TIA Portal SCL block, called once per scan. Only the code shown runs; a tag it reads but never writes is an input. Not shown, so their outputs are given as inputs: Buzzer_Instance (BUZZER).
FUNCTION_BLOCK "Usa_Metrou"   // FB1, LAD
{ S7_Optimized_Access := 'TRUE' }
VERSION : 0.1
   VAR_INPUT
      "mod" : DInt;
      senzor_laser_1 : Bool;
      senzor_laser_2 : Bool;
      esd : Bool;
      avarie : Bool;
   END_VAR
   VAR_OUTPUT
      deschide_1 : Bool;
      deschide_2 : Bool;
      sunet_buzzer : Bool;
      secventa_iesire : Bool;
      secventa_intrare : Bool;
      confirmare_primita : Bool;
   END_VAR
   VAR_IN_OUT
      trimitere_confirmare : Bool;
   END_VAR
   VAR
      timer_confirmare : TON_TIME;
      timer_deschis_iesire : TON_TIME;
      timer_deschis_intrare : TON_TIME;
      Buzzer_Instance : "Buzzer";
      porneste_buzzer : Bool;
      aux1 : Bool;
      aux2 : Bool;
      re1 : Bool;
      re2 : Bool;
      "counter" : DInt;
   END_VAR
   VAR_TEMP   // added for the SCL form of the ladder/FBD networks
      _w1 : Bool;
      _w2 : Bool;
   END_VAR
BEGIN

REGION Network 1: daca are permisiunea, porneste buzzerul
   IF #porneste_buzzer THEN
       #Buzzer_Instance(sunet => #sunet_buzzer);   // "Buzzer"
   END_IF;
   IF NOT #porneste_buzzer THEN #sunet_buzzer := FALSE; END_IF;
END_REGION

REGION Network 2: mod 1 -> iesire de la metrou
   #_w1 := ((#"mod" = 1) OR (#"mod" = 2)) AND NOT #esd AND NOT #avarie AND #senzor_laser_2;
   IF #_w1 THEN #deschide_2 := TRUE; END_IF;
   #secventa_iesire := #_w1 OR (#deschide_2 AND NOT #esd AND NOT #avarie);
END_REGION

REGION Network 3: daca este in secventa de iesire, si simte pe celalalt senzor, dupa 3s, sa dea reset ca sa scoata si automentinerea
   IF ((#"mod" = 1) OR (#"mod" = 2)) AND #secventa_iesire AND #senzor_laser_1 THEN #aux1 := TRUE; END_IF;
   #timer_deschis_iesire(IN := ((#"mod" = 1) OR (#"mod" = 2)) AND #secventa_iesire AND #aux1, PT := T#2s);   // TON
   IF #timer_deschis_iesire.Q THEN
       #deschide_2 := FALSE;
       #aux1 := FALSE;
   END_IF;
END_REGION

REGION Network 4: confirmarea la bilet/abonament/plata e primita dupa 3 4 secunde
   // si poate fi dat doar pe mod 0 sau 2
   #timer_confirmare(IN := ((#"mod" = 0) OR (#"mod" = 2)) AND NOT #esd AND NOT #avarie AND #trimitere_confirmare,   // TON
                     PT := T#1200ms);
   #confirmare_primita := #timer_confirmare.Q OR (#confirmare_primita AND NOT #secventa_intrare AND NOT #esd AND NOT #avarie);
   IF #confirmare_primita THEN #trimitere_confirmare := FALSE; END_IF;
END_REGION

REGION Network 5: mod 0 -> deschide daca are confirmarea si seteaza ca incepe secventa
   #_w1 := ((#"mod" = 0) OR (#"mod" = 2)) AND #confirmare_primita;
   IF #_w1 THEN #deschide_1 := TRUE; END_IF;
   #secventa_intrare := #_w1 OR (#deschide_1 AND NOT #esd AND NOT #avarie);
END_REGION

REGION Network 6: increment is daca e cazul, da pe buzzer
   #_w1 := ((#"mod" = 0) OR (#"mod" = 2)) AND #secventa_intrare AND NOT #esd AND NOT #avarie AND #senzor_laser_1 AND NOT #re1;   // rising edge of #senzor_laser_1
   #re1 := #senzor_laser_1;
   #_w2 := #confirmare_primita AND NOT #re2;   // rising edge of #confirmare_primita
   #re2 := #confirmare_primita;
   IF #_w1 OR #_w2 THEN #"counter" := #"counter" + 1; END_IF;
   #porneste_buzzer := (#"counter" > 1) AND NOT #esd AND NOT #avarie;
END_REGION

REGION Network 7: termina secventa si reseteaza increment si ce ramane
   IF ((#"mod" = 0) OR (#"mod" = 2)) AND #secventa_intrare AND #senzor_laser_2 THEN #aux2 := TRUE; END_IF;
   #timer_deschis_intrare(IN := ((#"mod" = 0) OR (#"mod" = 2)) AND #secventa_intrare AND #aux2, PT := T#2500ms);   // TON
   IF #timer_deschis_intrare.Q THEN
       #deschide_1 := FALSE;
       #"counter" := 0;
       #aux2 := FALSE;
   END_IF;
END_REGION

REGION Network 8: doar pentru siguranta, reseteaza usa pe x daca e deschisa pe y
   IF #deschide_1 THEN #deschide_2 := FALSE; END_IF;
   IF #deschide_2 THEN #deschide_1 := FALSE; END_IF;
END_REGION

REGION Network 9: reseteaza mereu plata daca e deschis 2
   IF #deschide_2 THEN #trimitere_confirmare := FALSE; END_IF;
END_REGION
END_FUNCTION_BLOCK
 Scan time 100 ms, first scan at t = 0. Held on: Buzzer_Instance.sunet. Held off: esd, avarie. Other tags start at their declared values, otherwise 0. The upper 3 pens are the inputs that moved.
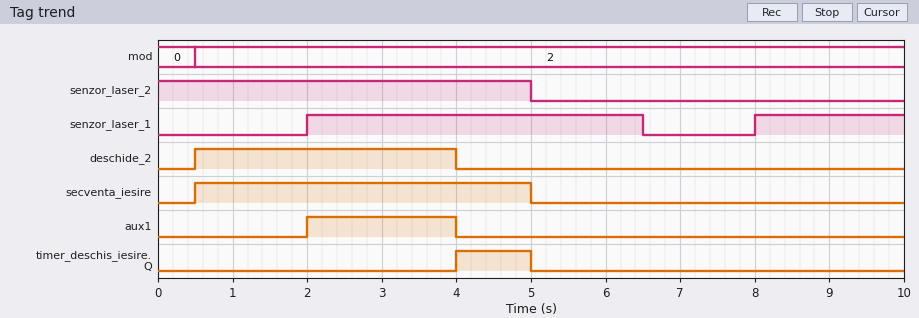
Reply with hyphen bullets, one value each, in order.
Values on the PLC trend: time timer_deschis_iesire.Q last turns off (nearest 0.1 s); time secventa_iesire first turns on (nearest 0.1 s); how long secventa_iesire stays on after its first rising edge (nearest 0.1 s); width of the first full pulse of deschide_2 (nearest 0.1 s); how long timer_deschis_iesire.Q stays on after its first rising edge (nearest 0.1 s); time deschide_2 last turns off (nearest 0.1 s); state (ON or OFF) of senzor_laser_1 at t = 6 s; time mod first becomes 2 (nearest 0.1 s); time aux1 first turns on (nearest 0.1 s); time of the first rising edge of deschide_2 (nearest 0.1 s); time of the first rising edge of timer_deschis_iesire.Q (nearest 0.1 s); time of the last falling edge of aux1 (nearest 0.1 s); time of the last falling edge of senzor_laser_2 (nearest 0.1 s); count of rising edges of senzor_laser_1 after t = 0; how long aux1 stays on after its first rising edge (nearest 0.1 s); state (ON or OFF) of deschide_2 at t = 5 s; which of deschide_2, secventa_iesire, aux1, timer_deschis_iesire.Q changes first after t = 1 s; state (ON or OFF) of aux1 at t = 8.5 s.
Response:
- 5.0 s
- 0.5 s
- 4.5 s
- 3.5 s
- 1.0 s
- 4.0 s
- ON
- 0.5 s
- 2.0 s
- 0.5 s
- 4.0 s
- 4.0 s
- 5.0 s
- 2
- 2.0 s
- OFF
- aux1
- OFF
